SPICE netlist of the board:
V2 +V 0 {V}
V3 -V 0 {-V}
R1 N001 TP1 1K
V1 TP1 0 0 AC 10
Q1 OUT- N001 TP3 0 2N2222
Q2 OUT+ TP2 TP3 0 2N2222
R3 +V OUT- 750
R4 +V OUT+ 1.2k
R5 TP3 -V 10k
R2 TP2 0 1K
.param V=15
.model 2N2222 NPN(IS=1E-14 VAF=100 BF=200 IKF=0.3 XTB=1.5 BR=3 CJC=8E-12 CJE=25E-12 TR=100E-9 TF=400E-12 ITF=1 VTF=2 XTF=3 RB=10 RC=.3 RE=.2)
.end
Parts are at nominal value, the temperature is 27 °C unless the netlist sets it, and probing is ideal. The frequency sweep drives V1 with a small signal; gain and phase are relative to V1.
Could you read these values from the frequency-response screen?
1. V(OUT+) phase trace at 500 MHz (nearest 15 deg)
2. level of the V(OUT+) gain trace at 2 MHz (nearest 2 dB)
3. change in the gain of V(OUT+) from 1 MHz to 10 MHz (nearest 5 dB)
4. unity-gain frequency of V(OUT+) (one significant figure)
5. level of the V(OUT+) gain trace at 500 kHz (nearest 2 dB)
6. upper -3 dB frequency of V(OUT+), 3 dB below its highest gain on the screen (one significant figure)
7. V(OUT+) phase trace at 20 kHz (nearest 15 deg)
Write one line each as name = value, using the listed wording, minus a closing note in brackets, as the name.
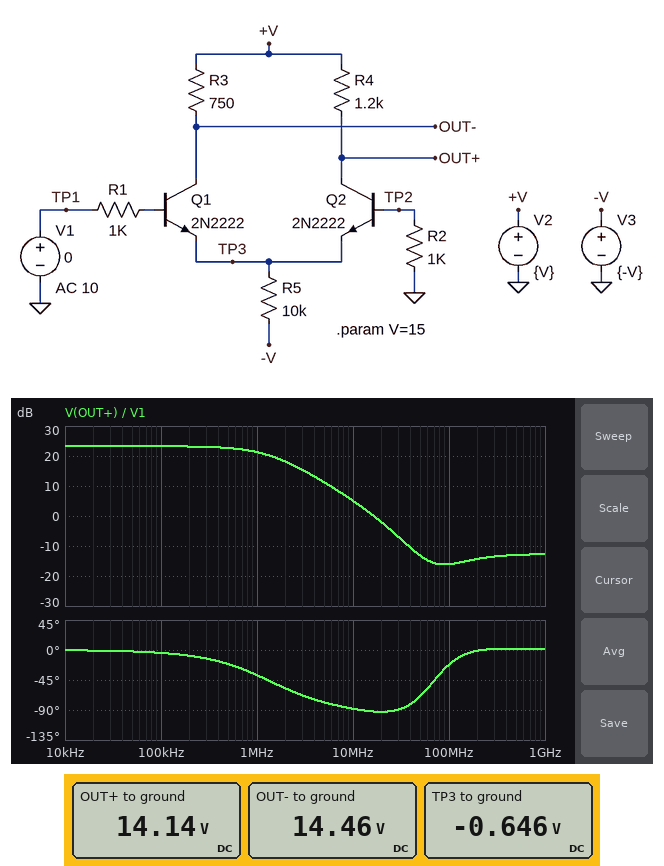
V(OUT+) phase trace at 500 MHz = 0 deg
level of the V(OUT+) gain trace at 2 MHz = 18 dB
change in the gain of V(OUT+) from 1 MHz to 10 MHz = -15 dB
unity-gain frequency of V(OUT+) = 20 MHz
level of the V(OUT+) gain trace at 500 kHz = 22 dB
upper -3 dB frequency of V(OUT+), 3 dB below its highest gain on the screen = 1 MHz
V(OUT+) phase trace at 20 kHz = 0 deg
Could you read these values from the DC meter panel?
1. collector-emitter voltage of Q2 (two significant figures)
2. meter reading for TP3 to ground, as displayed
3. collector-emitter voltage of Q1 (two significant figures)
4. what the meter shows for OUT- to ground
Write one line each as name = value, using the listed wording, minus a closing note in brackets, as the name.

collector-emitter voltage of Q2 = 15 V
meter reading for TP3 to ground, as displayed = -0.646 V
collector-emitter voltage of Q1 = 15 V
what the meter shows for OUT- to ground = 14.46 V
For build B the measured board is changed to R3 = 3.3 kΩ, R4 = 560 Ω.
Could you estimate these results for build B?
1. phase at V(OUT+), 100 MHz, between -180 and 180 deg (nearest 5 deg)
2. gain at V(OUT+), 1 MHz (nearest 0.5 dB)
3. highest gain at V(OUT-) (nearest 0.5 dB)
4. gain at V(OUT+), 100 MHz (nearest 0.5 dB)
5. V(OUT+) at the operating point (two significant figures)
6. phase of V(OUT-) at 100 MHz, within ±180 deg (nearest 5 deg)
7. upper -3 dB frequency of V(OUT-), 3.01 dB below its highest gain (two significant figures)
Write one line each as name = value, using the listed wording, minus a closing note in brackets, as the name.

phase at V(OUT+), 100 MHz, between -180 and 180 deg = 0 deg
gain at V(OUT+), 1 MHz = 12.5 dB
highest gain at V(OUT-) = 32.0 dB
gain at V(OUT+), 100 MHz = -17.0 dB
V(OUT+) at the operating point = 15 V
phase of V(OUT-) at 100 MHz, within ±180 deg = 20 deg
upper -3 dB frequency of V(OUT-), 3.01 dB below its highest gain = 800 kHz
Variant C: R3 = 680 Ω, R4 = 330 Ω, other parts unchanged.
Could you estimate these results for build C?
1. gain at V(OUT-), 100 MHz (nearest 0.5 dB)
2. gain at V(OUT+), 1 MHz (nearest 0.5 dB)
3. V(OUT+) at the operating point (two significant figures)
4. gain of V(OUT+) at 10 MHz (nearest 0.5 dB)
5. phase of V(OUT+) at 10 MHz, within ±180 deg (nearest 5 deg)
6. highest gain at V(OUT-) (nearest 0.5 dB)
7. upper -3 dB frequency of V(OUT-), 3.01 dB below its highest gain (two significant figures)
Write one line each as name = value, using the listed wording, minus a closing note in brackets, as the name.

gain at V(OUT-), 100 MHz = -11.0 dB
gain at V(OUT+), 1 MHz = 11.0 dB
V(OUT+) at the operating point = 15 V
gain of V(OUT+) at 10 MHz = -3.0 dB
phase of V(OUT+) at 10 MHz, within ±180 deg = -80 deg
highest gain at V(OUT-) = 18.5 dB
upper -3 dB frequency of V(OUT-), 3.01 dB below its highest gain = 1.9 MHz
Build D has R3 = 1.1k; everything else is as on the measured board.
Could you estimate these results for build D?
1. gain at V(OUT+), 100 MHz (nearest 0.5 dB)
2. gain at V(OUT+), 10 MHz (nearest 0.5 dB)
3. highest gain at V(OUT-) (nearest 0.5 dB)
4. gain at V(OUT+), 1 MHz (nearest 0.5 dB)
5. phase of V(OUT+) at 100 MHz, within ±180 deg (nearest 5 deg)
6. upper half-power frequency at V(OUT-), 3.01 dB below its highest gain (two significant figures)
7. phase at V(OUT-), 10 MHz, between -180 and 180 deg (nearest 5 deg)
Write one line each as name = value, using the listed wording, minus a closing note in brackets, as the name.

gain at V(OUT+), 100 MHz = -15.5 dB
gain at V(OUT+), 10 MHz = 4.0 dB
highest gain at V(OUT-) = 22.5 dB
gain at V(OUT+), 1 MHz = 21.0 dB
phase of V(OUT+) at 100 MHz, within ±180 deg = -15 deg
upper half-power frequency at V(OUT-), 3.01 dB below its highest gain = 1.2 MHz
phase at V(OUT-), 10 MHz, between -180 and 180 deg = 90 deg
